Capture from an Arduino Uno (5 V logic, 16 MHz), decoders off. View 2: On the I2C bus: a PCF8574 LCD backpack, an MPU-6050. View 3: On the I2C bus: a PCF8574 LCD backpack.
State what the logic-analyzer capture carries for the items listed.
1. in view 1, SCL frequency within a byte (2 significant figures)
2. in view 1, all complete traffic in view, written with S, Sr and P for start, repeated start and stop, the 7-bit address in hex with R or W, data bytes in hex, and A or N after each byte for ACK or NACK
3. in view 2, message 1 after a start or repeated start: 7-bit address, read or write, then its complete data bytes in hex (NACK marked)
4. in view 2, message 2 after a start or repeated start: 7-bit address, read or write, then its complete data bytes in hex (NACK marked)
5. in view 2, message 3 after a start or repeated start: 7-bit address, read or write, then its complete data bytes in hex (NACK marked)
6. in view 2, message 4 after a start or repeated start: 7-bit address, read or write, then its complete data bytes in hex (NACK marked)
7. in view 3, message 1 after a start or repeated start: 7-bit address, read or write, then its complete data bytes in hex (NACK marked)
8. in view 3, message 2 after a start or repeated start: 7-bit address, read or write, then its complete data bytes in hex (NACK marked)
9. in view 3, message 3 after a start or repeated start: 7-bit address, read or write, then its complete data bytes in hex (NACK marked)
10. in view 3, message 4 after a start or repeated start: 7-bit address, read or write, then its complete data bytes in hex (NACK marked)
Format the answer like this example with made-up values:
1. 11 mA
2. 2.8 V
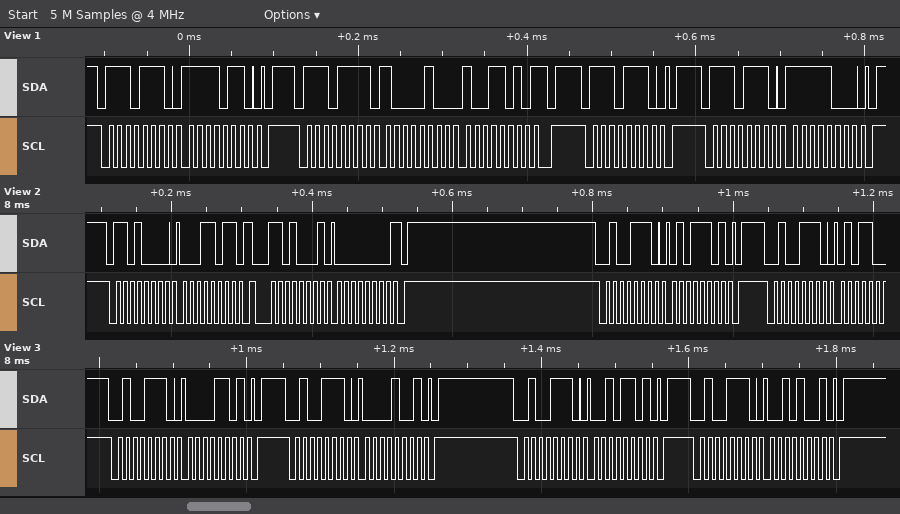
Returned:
1. 100 kHz
2. S 77W A F6 A P S 77R A 84 A 9A N P S 77W A P S 77W A F8 A P
3. 0x68 write: 1B
4. 0x68 read: 00 NACK
5. 0x27 write: 5D
6. 0x27 write
7. 0x27 write: 0D
8. 0x27 write: 09
9. 0x27 write: 2D
10. 0x27 write: 29
